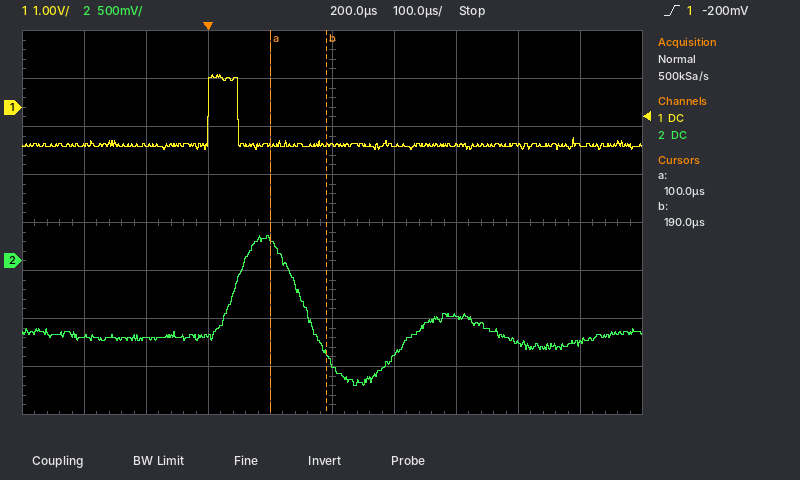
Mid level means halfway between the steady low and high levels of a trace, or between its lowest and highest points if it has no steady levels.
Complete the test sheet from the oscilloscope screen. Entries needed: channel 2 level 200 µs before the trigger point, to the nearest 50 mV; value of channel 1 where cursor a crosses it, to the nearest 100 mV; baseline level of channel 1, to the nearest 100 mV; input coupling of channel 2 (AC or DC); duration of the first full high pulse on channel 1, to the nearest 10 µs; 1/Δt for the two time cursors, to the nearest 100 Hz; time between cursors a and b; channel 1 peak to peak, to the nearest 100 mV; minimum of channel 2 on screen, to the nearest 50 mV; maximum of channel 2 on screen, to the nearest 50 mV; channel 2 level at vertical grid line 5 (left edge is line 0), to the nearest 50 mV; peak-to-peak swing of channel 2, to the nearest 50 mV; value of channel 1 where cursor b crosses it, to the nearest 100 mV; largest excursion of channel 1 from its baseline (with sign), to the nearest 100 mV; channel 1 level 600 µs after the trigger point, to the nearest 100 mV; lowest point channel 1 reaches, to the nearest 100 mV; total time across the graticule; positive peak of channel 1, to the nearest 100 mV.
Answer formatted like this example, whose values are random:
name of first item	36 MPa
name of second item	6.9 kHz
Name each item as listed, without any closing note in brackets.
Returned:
channel 2 level 200 µs before the trigger point, to the nearest 50 mV	-800 mV
value of channel 1 where cursor a crosses it, to the nearest 100 mV	-800 mV
baseline level of channel 1, to the nearest 100 mV	-800 mV
input coupling of channel 2	DC
duration of the first full high pulse on channel 1, to the nearest 10 µs	50 µs
1/Δt for the two time cursors, to the nearest 100 Hz	11.1 kHz
time between cursors a and b	90 µs
channel 1 peak to peak, to the nearest 100 mV	1.6 V
minimum of channel 2 on screen, to the nearest 50 mV	-1.30 V
maximum of channel 2 on screen, to the nearest 50 mV	250 mV
channel 2 level at vertical grid line 5 (left edge is line 0), to the nearest 50 mV	-1.05 V
peak-to-peak swing of channel 2, to the nearest 50 mV	1.55 V
value of channel 1 where cursor b crosses it, to the nearest 100 mV	-800 mV
largest excursion of channel 1 from its baseline (with sign), to the nearest 100 mV	+1.5 V
channel 1 level 600 µs after the trigger point, to the nearest 100 mV	-800 mV
lowest point channel 1 reaches, to the nearest 100 mV	-900 mV
total time across the graticule	1 ms
positive peak of channel 1, to the nearest 100 mV	700 mV
